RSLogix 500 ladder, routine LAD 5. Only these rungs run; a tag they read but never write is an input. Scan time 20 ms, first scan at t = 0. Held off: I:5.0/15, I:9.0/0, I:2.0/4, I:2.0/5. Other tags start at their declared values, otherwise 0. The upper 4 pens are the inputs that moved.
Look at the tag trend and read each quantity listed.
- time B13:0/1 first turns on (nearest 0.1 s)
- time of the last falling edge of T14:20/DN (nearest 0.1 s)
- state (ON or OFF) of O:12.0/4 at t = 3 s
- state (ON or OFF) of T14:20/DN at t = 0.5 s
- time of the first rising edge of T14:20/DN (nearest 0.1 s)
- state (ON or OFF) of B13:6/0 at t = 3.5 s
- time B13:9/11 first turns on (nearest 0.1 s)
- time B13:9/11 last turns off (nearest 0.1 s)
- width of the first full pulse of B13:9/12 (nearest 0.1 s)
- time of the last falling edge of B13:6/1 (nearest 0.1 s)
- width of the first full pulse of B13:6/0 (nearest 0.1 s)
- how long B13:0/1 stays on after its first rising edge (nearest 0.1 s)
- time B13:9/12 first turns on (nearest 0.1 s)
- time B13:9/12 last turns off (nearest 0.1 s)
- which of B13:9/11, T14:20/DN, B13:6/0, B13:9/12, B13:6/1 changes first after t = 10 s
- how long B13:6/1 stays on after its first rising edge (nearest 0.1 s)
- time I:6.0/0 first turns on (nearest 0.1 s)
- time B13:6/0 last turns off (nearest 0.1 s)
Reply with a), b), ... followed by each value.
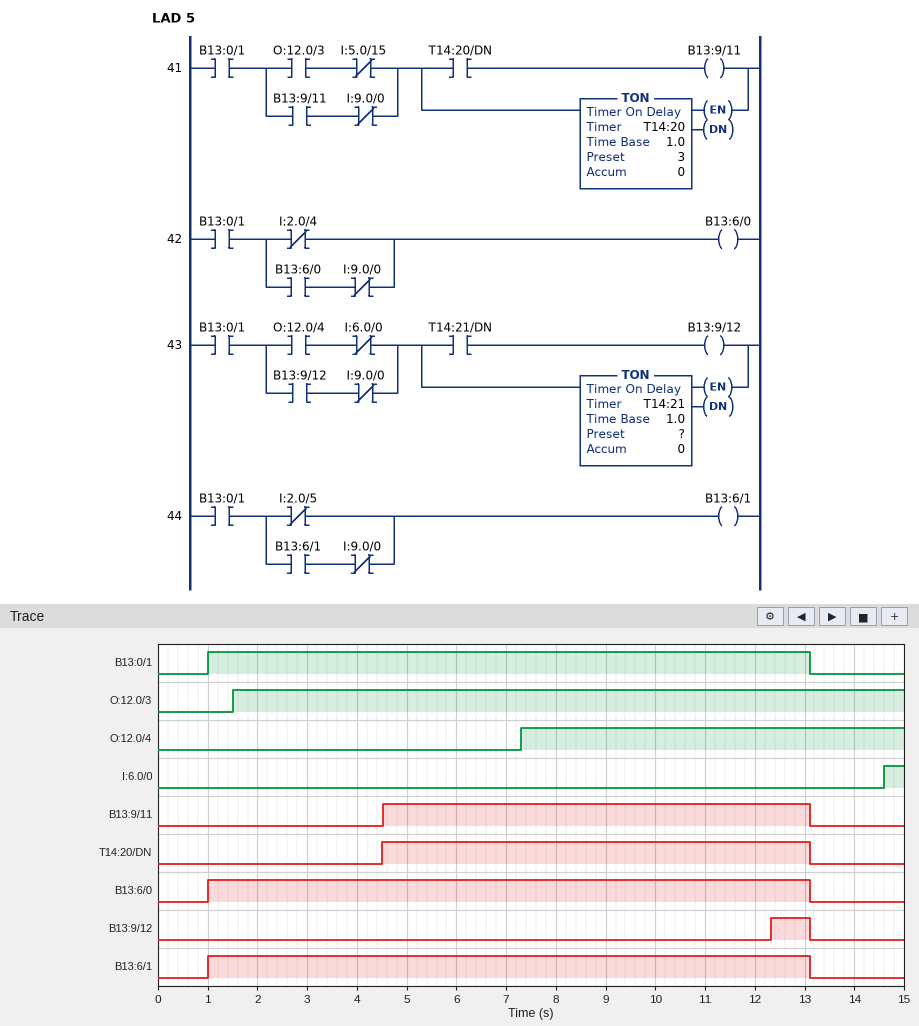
a) 1.0 s
b) 13.1 s
c) OFF
d) OFF
e) 4.5 s
f) ON
g) 4.5 s
h) 13.1 s
i) 0.8 s
j) 13.1 s
k) 12.1 s
l) 12.1 s
m) 12.3 s
n) 13.1 s
o) B13:9/12
p) 12.1 s
q) 14.6 s
r) 13.1 s
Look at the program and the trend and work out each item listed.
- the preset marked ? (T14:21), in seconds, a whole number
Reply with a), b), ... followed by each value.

a) 5 s
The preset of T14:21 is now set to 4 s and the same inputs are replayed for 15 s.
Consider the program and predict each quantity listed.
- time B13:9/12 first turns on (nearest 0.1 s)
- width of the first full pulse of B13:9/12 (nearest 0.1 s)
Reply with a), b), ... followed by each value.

a) 11.3 s
b) 1.8 s
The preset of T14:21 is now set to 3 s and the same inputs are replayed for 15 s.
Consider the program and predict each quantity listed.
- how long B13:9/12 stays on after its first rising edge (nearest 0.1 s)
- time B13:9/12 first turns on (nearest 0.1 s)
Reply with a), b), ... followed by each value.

a) 2.8 s
b) 10.3 s
